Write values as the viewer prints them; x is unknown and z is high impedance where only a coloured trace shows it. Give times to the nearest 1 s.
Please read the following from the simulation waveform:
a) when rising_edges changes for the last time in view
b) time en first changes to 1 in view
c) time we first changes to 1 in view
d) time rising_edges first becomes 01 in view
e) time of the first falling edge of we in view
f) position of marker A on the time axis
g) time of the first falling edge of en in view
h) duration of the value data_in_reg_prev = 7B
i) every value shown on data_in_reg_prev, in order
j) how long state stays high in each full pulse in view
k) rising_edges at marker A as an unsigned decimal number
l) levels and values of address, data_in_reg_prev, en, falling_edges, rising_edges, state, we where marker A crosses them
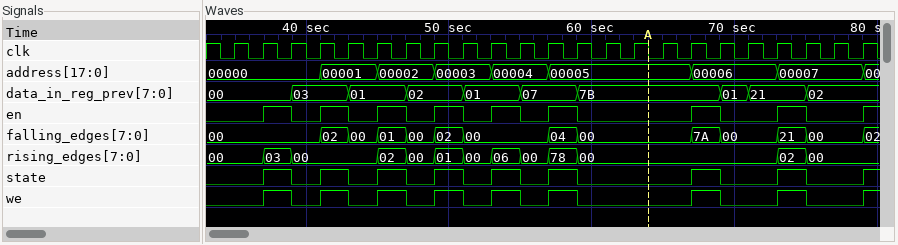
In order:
75 s
37 s
37 s
49 s
39 s
64 s
39 s
10 s
00, 03, 01, 02, 01, 07, 7B, 01, 21, 02
2 s, 2 s, 2 s, 2 s, 2 s, 2 s, 2 s, 2 s
0
address=00005, data_in_reg_prev=7B, en=0, falling_edges=00, rising_edges=00, state=0, we=0
